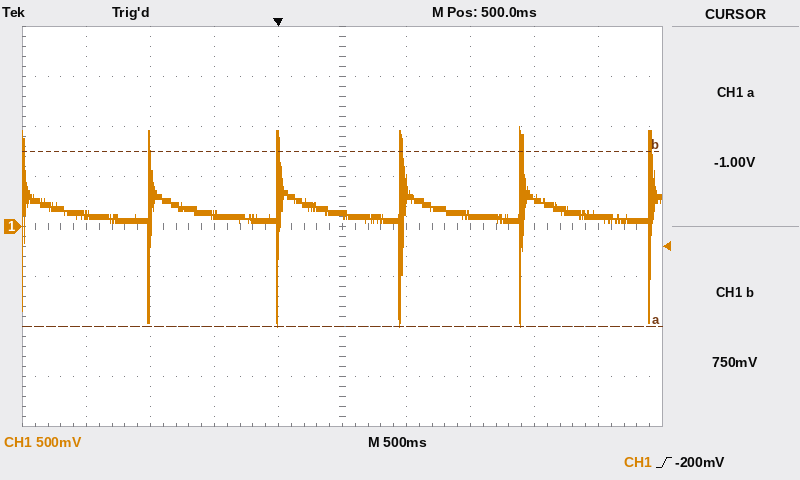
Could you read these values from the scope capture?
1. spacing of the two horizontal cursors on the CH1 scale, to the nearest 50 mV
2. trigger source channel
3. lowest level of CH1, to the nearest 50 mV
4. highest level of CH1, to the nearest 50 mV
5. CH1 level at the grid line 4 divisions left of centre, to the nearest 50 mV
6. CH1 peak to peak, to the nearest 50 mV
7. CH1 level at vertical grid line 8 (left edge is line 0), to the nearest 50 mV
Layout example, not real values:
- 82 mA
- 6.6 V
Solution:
- 1.75 V
- CH1
- -1.00 V
- 1.00 V
- 100 mV
- 2.00 V
- 300 mV
